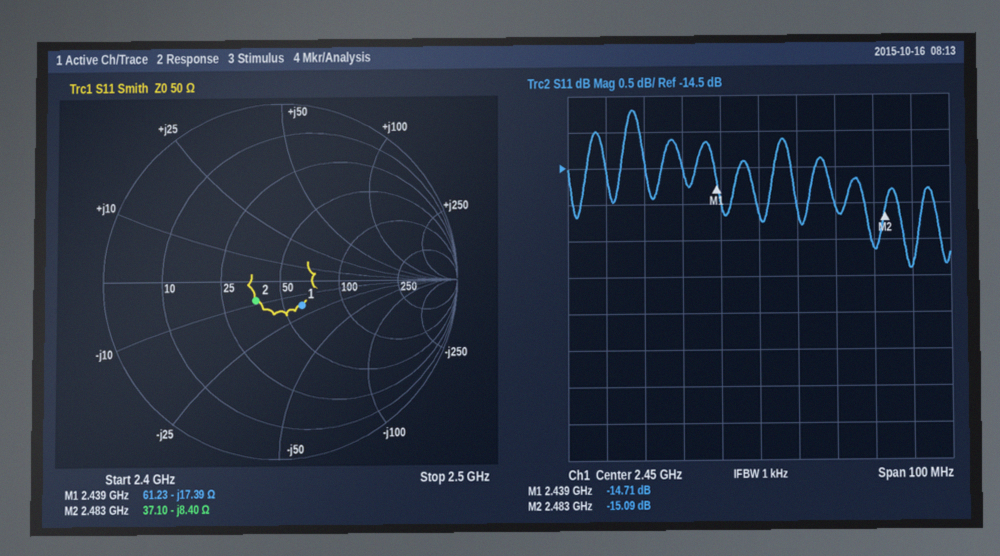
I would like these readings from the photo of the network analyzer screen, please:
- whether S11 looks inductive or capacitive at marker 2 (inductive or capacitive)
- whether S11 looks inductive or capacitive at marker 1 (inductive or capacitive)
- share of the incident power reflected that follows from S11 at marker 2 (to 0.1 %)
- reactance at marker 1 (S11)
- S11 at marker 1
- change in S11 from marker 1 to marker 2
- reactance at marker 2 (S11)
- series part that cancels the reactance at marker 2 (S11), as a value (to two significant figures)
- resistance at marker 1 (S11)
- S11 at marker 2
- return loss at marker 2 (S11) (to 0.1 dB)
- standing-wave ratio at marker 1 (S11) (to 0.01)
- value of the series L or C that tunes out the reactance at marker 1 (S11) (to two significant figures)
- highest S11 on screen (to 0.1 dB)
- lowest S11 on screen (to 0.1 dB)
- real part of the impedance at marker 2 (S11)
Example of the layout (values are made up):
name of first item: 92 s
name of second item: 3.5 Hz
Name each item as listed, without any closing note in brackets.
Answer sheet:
whether S11 looks inductive or capacitive at marker 2: capacitive
whether S11 looks inductive or capacitive at marker 1: capacitive
share of the incident power reflected that follows from S11 at marker 2: 3.1 %
reactance at marker 1: -17.39 Ω
S11 at marker 1: -14.71 dB
change in S11 from marker 1 to marker 2: -0.38 dB
reactance at marker 2: -8.40 Ω
series part that cancels the reactance at marker 2 (S11), as a value: 540 pH
resistance at marker 1: 61.23 Ω
S11 at marker 2: -15.09 dB
return loss at marker 2 (S11): 15.1 dB
standing-wave ratio at marker 1 (S11): 1.45
value of the series L or C that tunes out the reactance at marker 1 (S11): 1.1 nH
highest S11 on screen: -13.7 dB
lowest S11 on screen: -15.9 dB
real part of the impedance at marker 2: 37.10 Ω
